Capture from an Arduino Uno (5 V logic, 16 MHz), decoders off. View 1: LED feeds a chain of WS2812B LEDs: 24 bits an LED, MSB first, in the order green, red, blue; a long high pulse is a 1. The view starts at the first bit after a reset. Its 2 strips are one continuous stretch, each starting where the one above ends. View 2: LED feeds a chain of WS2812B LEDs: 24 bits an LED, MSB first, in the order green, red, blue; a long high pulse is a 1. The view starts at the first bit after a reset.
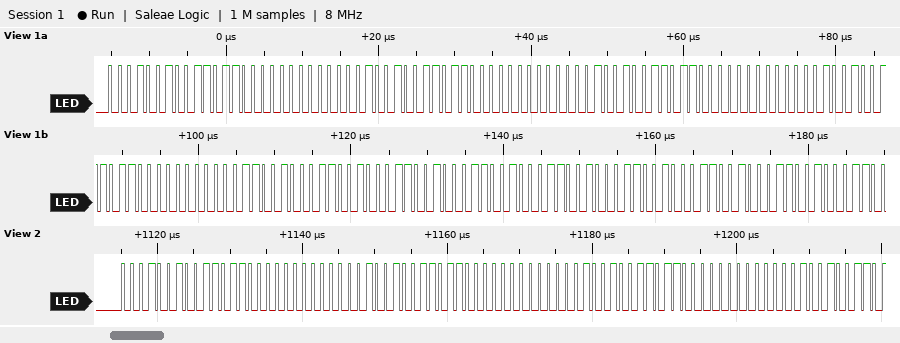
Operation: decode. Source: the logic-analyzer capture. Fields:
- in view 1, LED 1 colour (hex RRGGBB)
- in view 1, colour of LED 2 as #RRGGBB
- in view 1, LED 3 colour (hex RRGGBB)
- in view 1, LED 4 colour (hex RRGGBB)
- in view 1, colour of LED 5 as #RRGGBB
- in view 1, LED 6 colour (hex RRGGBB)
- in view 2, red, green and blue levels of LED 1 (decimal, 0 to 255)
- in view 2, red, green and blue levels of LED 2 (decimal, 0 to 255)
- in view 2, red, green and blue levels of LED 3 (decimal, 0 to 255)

#6C1200
#6C1200
#6C1200
#6C1200
#646464
#646464
108, 18, 0
108, 18, 0
108, 18, 0
